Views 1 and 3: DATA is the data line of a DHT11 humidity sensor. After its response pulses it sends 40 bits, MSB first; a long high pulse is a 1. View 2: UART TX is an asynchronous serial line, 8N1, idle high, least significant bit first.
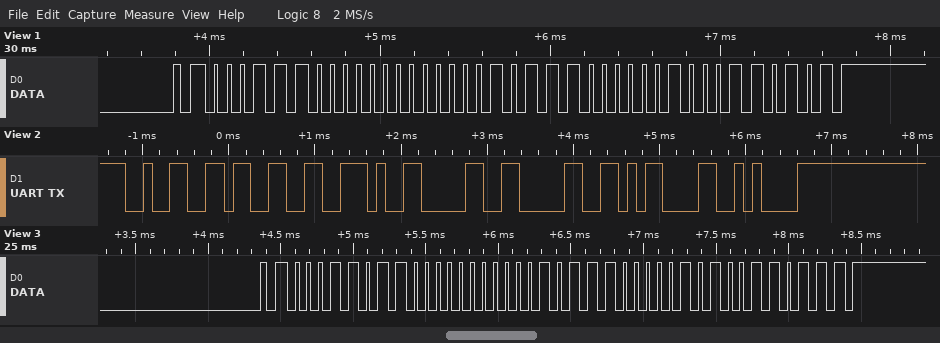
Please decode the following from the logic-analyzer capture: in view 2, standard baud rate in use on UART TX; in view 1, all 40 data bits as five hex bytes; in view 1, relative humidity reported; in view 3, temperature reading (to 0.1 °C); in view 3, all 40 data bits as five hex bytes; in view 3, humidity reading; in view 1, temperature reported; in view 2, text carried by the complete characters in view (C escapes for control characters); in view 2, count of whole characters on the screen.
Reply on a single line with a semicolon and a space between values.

9600 baud; 1C 00 17 02 35; 28 %; 23.5 °C; 1B 00 17 05 37; 27 %; 23.2 °C; "23.00\r\n"; 7
